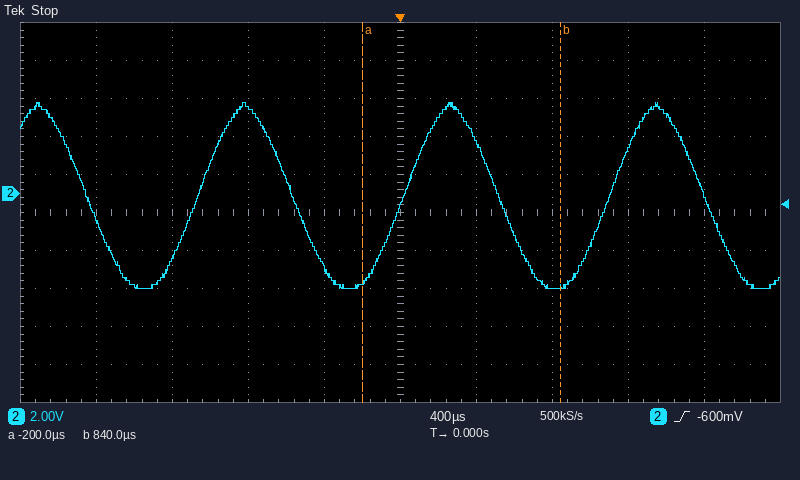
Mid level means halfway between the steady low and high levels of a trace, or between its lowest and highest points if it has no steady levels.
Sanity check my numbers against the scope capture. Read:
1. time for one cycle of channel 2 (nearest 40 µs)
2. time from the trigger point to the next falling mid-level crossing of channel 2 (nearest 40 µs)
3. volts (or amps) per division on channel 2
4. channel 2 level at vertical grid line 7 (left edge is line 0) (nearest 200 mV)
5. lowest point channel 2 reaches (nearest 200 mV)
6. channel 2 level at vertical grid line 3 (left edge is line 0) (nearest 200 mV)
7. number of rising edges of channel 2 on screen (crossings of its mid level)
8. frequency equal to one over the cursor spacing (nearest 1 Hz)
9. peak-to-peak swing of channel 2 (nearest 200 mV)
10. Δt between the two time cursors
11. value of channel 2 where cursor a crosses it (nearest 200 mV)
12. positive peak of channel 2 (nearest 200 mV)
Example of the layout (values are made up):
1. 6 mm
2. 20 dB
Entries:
1. 1.08 ms
2. 520 µs
3. 2 V
4. -5.0 V
5. -5.0 V
6. 4.6 V
7. 3
8. 962 Hz
9. 9.8 V
10. 1.04 ms
11. -4.6 V
12. 4.8 V
